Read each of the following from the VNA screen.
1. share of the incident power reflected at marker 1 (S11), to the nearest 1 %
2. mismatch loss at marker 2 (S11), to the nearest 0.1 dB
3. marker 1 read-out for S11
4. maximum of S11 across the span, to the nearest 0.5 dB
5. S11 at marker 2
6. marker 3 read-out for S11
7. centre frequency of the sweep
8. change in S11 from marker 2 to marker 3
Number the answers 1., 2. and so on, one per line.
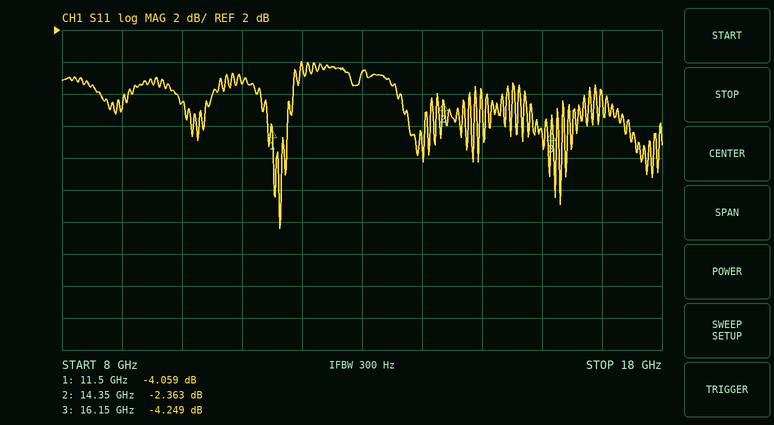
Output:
1. 39 %
2. 3.8 dB
3. -4.059 dB
4. 0.0 dB
5. -2.363 dB
6. -4.249 dB
7. 13 GHz
8. -1.886 dB
